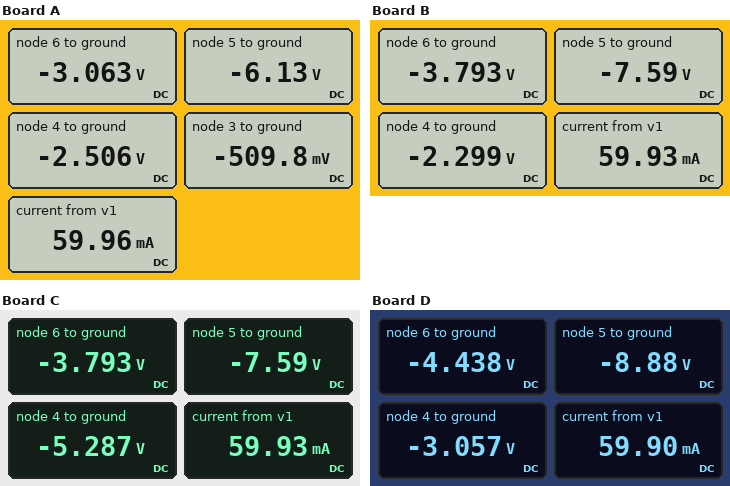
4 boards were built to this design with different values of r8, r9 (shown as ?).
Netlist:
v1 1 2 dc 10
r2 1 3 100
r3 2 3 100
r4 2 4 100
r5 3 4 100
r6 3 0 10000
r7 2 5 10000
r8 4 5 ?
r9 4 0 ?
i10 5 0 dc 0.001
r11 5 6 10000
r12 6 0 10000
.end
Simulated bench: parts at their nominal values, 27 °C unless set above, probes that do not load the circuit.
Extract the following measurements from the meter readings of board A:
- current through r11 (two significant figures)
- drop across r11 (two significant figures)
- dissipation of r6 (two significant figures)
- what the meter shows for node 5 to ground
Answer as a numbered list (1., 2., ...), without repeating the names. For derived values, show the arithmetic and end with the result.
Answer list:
1. (-3.063 V - (-6.13 V)) / 10 kΩ = 310 µA
2. -3.063 V - (-6.13 V) = 3.1 V
3. (0 V - (-509.8 mV))^2 / 10 kΩ = 26 µW
4. -6.13 V
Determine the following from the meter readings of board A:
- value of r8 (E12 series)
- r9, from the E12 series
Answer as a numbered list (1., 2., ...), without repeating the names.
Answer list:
1. 6.8 kΩ
2. 3.9 kΩ
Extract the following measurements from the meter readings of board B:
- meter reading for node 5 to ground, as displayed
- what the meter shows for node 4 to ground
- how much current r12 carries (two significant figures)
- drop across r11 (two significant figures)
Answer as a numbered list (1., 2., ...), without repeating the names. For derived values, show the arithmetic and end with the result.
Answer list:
1. -7.59 V
2. -2.299 V
3. (0 V - (-3.793 V)) / 10 kΩ = 380 µA
4. -3.793 V - (-7.59 V) = 3.8 V
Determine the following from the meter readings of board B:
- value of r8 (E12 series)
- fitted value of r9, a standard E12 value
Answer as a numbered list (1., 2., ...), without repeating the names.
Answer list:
1. 18 kΩ
2. 3.9 kΩ
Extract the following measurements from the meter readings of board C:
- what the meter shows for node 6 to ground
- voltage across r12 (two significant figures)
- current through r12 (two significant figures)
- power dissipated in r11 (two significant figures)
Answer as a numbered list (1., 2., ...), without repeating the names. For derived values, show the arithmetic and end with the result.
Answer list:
1. -3.793 V
2. 0 V - (-3.793 V) = 3.8 V
3. (0 V - (-3.793 V)) / 10 kΩ = 380 µA
4. (-3.793 V - (-7.59 V))^2 / 10 kΩ = 1.4 mW
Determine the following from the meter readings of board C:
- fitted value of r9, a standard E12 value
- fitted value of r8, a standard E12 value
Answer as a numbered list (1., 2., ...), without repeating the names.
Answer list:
1. 18 kΩ
2. 3.9 kΩ
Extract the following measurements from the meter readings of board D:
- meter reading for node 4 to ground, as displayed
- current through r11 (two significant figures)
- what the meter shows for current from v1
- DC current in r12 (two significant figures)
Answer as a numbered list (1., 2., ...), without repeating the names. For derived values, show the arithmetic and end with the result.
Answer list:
1. -3.057 V
2. (-4.438 V - (-8.88 V)) / 10 kΩ = 440 µA
3. 59.90 mA
4. (0 V - (-4.438 V)) / 10 kΩ = 440 µA
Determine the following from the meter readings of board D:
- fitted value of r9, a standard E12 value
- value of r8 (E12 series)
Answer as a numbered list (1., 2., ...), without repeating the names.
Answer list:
1. 6.8 kΩ
2. 33 kΩ
